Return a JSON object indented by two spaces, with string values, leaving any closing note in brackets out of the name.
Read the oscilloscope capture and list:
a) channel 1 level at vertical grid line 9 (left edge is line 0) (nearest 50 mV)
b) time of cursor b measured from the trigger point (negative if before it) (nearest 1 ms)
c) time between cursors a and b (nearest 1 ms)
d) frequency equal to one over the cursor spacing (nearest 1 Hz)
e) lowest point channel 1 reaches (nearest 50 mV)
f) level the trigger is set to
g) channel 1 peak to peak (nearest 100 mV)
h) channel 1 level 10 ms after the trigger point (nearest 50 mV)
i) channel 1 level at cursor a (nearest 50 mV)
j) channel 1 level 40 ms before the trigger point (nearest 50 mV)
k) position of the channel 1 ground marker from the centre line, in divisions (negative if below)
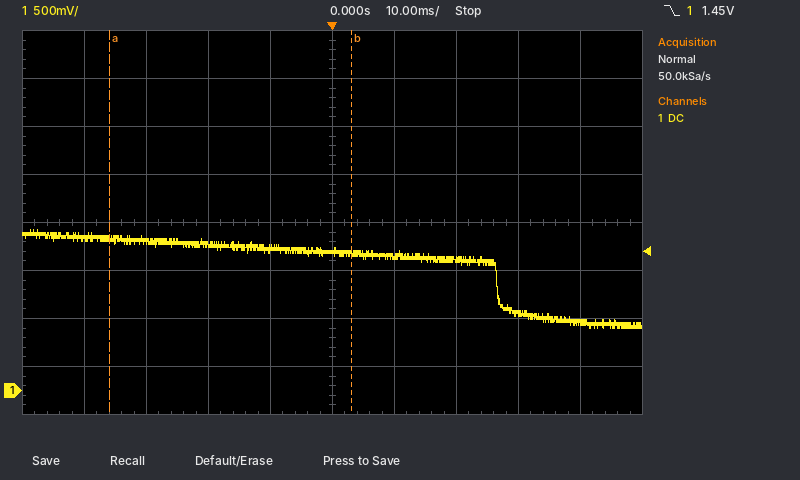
{
  "channel 1 level at vertical grid line 9 (left edge is line 0)": "700 mV",
  "time of cursor b measured from the trigger point (negative if before it)": "+3 ms",
  "time between cursors a and b": "39 ms",
  "frequency equal to one over the cursor spacing": "26 Hz",
  "lowest point channel 1 reaches": "650 mV",
  "level the trigger is set to": "1.45 V",
  "channel 1 peak to peak": "1.00 V",
  "channel 1 level 10 ms after the trigger point": "1.40 V",
  "channel 1 level at cursor a": "1.60 V",
  "channel 1 level 40 ms before the trigger point": "1.60 V",
  "position of the channel 1 ground marker from the centre line, in divisions": "-3.5 div"
}
